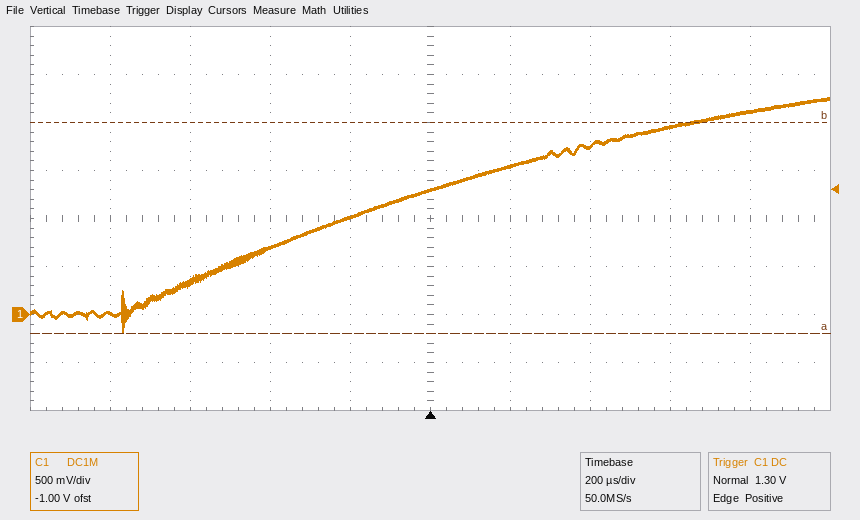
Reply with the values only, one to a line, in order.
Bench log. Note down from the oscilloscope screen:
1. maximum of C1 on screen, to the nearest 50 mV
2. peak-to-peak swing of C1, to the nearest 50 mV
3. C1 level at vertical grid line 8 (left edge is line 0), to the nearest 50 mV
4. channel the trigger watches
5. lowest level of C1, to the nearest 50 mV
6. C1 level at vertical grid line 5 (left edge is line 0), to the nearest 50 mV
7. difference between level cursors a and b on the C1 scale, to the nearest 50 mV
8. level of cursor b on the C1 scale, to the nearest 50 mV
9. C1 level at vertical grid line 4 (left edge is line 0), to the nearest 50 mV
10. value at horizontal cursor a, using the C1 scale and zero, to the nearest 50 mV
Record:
2.25 V
2.45 V
1.95 V
C1
-200 mV
1.30 V
2.20 V
2.00 V
1.00 V
-200 mV
